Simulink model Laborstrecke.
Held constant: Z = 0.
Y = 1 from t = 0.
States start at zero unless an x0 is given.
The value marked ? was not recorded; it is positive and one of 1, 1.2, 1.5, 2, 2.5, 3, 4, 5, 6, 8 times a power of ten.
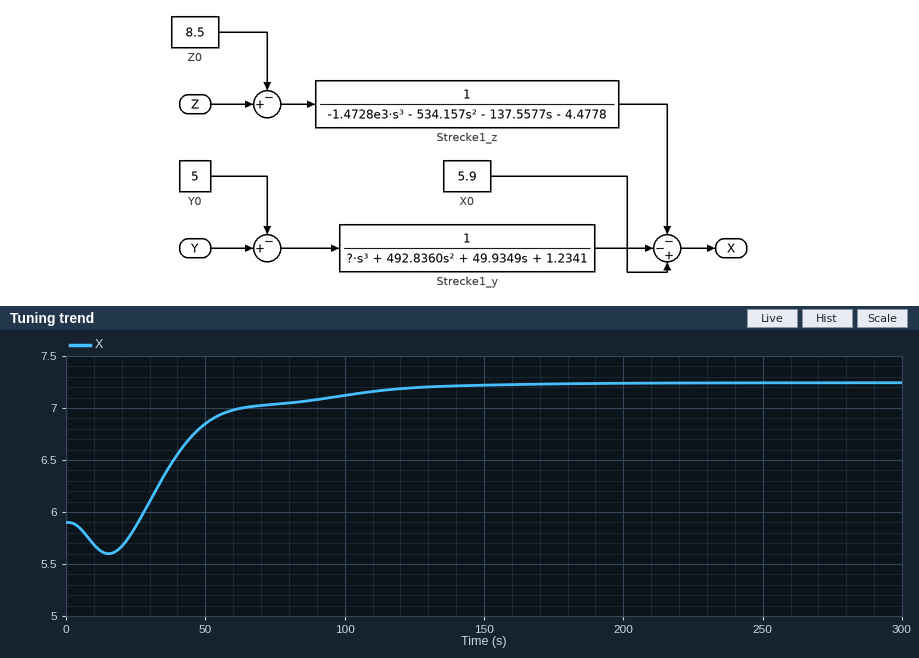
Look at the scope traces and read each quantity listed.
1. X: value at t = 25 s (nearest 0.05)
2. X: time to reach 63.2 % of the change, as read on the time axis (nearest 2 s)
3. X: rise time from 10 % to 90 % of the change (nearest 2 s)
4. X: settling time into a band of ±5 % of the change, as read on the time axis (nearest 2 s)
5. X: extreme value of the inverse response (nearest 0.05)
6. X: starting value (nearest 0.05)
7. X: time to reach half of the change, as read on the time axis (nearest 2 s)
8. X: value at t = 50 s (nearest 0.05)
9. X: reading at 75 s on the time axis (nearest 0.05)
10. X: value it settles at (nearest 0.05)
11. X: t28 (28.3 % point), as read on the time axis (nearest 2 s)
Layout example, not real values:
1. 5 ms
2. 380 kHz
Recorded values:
1. 5.85
2. 46 s
3. 68 s
4. 116 s
5. 5.60
6. 5.90
7. 40 s
8. 6.85
9. 7.05
10. 7.25
11. 34 s
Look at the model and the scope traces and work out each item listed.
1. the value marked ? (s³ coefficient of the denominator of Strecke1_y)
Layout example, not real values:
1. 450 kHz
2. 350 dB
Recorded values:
1. 4000
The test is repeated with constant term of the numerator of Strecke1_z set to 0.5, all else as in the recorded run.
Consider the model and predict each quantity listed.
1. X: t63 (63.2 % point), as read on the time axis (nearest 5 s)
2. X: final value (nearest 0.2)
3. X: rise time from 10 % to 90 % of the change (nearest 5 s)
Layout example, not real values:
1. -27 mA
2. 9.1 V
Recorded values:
1. 40 s
2. 8.2
3. 65 s
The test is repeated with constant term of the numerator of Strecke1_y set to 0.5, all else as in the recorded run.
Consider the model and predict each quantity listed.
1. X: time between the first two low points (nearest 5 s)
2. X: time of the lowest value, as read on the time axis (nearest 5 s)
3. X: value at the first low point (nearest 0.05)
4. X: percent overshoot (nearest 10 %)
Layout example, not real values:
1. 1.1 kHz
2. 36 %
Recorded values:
1. 65 s
2. 20 s
3. 5.35
4. 100 %
